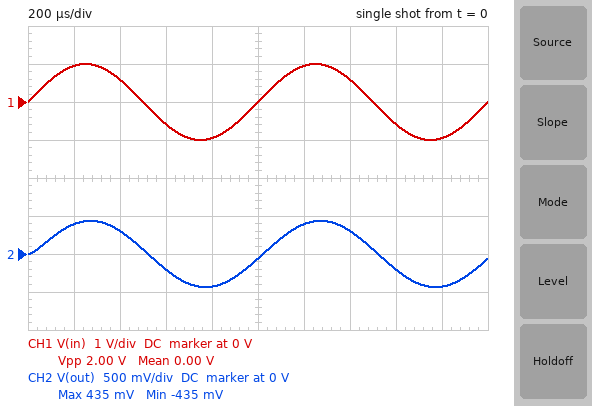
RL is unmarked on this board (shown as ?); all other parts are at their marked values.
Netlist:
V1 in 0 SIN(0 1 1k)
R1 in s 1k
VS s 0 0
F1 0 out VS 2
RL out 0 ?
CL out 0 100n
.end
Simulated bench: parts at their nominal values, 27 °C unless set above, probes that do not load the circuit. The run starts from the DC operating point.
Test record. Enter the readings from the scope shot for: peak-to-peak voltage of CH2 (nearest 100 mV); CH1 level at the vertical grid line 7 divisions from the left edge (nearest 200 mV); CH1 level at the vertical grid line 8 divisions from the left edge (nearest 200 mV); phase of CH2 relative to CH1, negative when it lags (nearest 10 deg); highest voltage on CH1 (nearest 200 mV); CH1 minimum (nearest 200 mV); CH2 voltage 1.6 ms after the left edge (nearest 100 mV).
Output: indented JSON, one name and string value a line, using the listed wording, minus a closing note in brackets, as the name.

{
  "peak-to-peak voltage of CH2": "900 mV",
  "CH1 level at the vertical grid line 7 divisions from the left edge": "600 mV",
  "CH1 level at the vertical grid line 8 divisions from the left edge": "-600 mV",
  "phase of CH2 relative to CH1, negative when it lags": "-10 deg",
  "highest voltage on CH1": "1.0 V",
  "CH1 minimum": "-1.0 V",
  "CH2 voltage 1.6 ms after the left edge": "-200 mV"
}
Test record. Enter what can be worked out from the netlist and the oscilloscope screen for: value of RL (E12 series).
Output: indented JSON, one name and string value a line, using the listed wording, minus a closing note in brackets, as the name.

{
  "value of RL": "220 Ω"
}
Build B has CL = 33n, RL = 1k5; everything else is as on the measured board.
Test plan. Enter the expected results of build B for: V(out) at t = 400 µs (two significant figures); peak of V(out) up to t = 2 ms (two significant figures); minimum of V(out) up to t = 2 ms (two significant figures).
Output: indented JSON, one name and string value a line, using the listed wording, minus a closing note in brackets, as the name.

{
  "V(out) at t = 400 µs": "2.3 V",
  "peak of V(out) up to t = 2 ms": "2.9 V",
  "minimum of V(out) up to t = 2 ms": "-2.9 V"
}
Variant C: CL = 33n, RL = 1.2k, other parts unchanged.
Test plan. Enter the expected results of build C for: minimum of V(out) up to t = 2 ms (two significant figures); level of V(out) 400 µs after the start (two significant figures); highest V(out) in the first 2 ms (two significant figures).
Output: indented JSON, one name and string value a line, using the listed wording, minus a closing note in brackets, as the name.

{
  "minimum of V(out) up to t = 2 ms": "-2.3 V",
  "level of V(out) 400 µs after the start": "1.8 V",
  "highest V(out) in the first 2 ms": "2.3 V"
}
